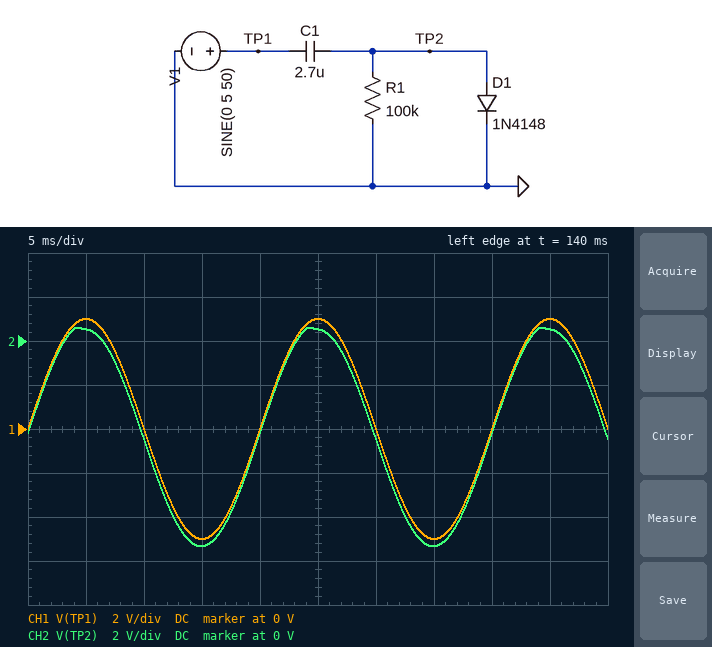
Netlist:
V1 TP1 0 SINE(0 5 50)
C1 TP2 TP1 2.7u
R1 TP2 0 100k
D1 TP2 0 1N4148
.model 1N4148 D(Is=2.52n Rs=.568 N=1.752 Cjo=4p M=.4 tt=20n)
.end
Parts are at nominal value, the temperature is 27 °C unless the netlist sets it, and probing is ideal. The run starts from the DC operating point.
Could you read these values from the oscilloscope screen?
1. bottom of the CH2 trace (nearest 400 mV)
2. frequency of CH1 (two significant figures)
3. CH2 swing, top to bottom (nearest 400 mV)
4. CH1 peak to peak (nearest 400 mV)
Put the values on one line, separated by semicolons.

-9.2 V; 50 Hz; 10.0 V; 10.0 V
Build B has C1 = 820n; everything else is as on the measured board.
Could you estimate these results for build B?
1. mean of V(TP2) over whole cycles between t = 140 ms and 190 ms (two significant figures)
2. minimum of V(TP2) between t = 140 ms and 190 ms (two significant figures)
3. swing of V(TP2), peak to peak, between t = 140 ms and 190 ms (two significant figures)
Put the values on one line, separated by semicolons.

-4.1 V; -9.0 V; 9.6 V
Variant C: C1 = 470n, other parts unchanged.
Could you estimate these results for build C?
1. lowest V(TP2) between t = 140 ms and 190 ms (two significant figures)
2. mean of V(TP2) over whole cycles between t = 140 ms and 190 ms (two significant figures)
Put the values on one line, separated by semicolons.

-8.7 V; -3.8 V
